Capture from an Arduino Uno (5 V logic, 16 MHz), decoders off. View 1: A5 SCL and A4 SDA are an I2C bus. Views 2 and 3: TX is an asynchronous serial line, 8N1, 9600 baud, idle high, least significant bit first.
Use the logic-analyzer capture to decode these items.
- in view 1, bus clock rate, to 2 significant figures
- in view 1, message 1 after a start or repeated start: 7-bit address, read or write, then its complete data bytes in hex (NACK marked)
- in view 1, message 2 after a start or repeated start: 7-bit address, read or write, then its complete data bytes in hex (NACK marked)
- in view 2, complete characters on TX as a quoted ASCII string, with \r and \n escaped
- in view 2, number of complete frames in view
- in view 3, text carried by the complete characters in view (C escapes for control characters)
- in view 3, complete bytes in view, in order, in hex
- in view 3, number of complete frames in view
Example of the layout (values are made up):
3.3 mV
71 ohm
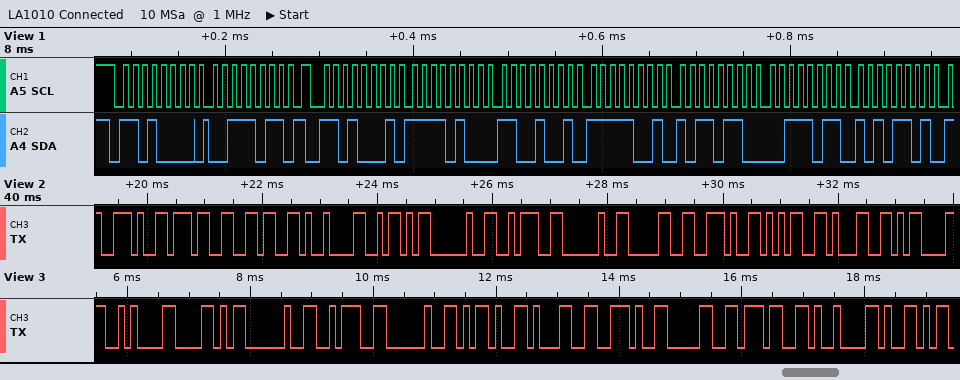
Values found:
100 kHz
0x68 write: 3B
0x68 read: F4 C9 F9 B6 3B AD
".76\tZ : 0.51\r"
13
"\nX : -1.07\tY"
0x0A 0x58 0x20 0x3A 0x20 0x2D 0x31 0x2E 0x30 0x37 0x09 0x59
12
